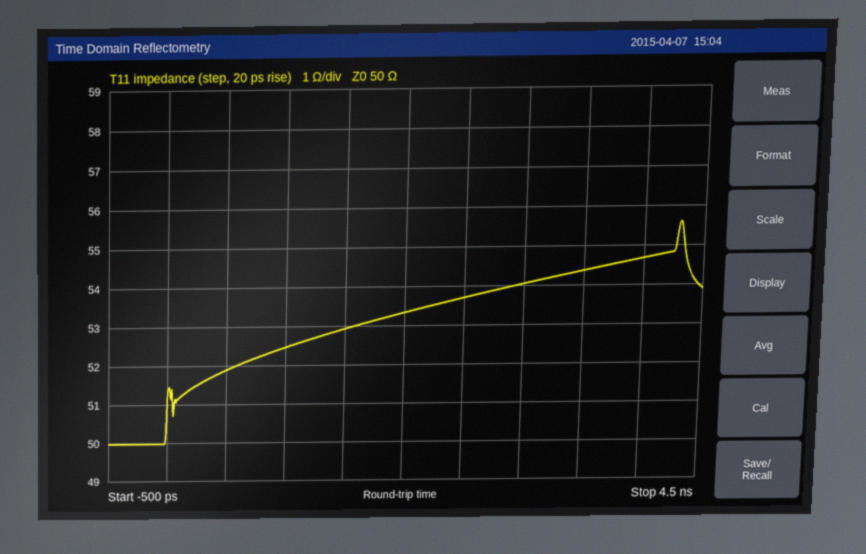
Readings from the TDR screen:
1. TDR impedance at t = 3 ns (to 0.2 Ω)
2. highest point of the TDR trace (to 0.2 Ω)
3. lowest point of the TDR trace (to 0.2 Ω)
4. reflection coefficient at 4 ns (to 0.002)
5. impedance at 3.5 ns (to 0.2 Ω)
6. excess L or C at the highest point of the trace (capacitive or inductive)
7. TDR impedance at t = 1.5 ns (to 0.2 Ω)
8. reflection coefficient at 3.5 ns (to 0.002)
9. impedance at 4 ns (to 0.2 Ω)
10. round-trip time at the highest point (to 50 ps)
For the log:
54.0 Ω
55.6 Ω
50.0 Ω
+0.044
54.4 Ω
inductive
53.0 Ω
+0.042
54.6 Ω
4.30 ns
